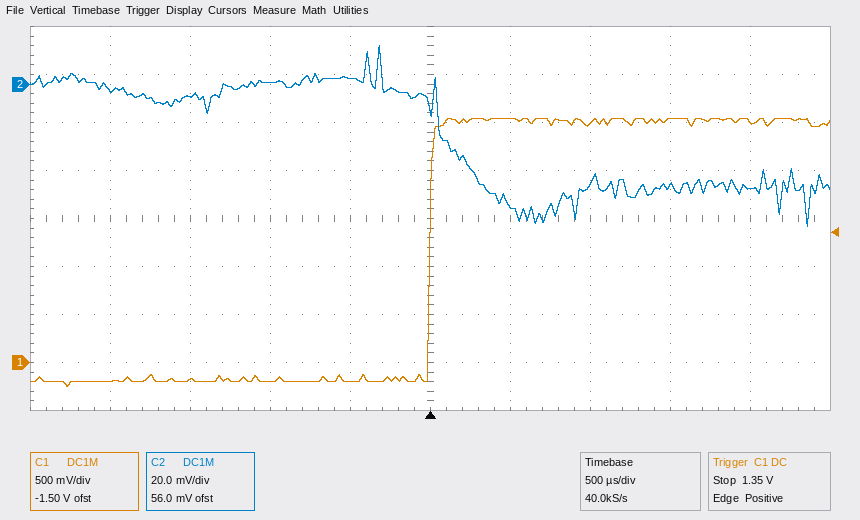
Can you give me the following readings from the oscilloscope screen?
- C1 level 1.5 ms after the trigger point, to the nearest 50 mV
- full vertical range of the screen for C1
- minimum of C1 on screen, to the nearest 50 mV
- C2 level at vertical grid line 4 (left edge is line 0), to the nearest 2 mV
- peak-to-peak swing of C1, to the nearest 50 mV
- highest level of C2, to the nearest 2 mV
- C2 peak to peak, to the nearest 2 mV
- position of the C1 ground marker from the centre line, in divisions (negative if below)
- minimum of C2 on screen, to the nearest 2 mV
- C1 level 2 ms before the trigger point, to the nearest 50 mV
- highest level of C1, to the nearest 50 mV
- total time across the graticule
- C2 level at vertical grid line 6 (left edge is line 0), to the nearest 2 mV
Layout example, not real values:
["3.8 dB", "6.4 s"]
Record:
["2.55 V", "4 V", "-250 mV", "2 mV", "2.80 V", "16 mV", "76 mV", "-3.0 div", "-60 mV", "-200 mV", "2.55 V", "5 ms", "-50 mV"]
